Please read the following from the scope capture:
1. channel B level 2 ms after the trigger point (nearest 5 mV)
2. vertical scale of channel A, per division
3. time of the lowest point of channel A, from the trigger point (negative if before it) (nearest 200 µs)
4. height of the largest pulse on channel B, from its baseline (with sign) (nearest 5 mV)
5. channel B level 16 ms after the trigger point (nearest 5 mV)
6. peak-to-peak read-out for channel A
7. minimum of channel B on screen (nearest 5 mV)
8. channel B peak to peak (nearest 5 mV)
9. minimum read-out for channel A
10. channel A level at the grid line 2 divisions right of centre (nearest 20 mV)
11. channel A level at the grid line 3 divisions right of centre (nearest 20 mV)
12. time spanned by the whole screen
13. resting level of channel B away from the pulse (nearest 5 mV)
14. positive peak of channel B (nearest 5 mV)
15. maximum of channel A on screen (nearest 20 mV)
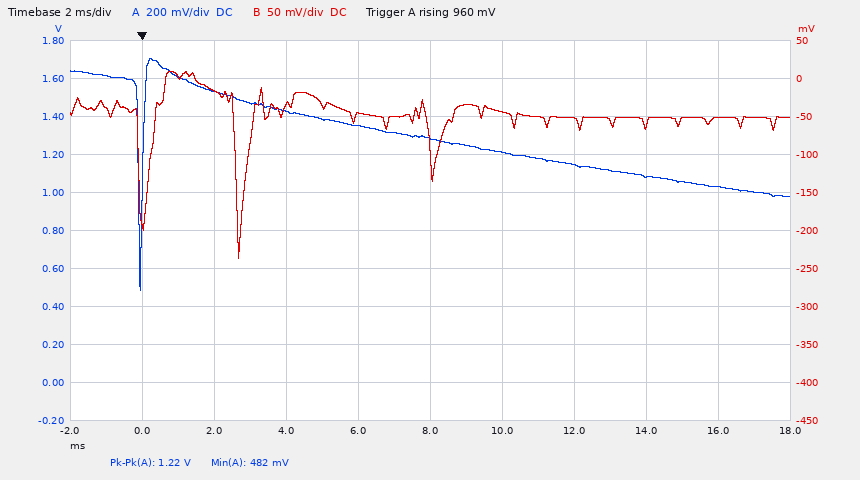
-15 mV
200 mV
0.0 ms
-185 mV
-50 mV
1.22 V
-235 mV
245 mV
482 mV
1.14 V
1.08 V
20 ms
-50 mV
10 mV
1.70 V
